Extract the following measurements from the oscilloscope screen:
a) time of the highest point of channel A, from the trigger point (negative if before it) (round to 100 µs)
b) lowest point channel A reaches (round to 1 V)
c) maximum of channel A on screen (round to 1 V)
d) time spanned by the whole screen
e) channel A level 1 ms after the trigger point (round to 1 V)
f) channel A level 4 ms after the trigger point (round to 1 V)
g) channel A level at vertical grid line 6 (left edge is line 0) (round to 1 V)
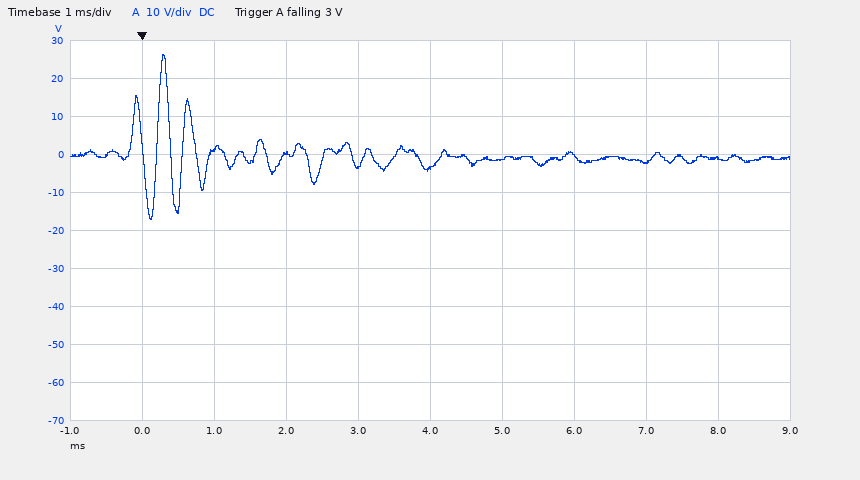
+300 µs
-17 V
26 V
10 ms
2 V
-4 V
-1 V
